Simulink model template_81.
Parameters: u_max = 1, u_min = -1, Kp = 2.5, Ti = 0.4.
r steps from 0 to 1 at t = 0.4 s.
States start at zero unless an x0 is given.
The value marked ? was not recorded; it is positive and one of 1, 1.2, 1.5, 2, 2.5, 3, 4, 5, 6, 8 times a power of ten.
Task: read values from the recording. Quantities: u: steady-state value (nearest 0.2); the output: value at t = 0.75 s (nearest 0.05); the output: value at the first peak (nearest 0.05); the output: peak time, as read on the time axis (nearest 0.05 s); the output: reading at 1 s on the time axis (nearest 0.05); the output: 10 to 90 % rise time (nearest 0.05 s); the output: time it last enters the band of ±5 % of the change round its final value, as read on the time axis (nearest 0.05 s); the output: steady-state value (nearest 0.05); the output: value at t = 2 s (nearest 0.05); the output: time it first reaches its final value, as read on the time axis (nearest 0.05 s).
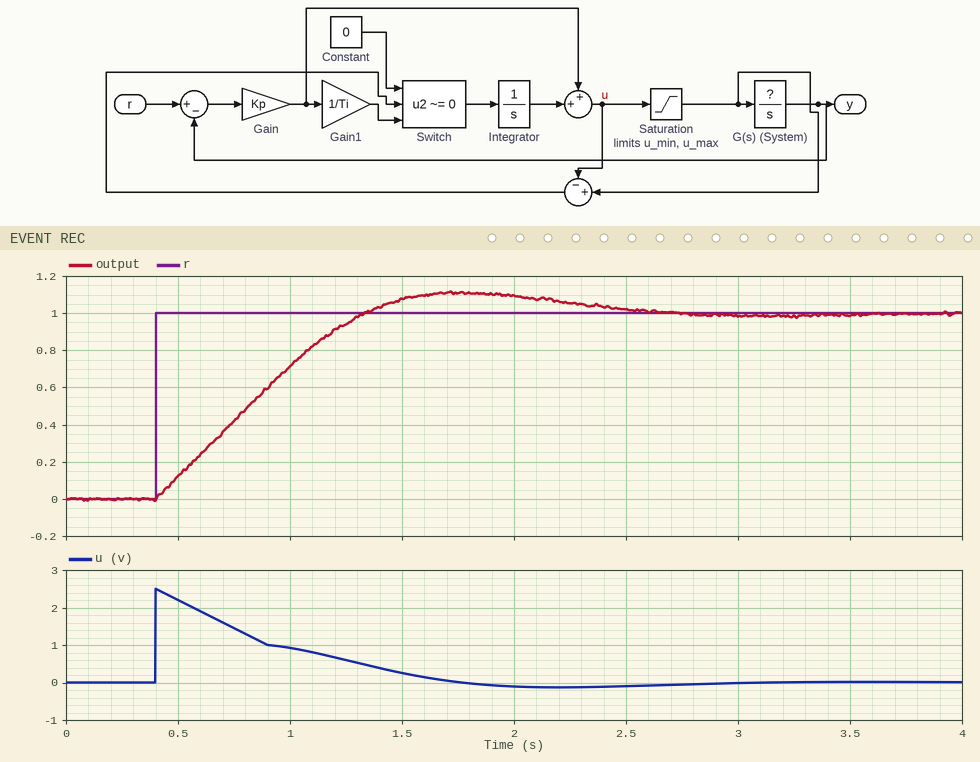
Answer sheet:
0.0
0.40
1.10
1.75 s
0.70
0.70 s
2.30 s
1.00
1.10
1.35 s
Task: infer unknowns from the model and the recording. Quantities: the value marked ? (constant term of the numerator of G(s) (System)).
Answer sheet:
1.2
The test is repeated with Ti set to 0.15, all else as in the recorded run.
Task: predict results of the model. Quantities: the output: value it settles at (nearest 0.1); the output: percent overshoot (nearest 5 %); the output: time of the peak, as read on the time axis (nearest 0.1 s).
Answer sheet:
1.0
15 %
1.5 s
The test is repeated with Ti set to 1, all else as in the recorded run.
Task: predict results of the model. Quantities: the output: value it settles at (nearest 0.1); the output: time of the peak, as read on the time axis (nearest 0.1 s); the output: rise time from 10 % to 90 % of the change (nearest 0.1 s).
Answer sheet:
1.0
2.1 s
0.8 s
